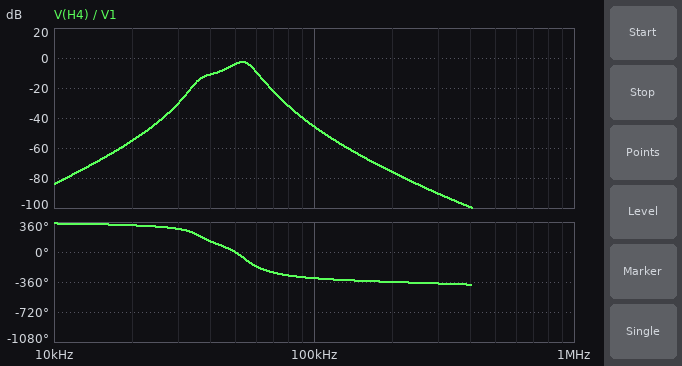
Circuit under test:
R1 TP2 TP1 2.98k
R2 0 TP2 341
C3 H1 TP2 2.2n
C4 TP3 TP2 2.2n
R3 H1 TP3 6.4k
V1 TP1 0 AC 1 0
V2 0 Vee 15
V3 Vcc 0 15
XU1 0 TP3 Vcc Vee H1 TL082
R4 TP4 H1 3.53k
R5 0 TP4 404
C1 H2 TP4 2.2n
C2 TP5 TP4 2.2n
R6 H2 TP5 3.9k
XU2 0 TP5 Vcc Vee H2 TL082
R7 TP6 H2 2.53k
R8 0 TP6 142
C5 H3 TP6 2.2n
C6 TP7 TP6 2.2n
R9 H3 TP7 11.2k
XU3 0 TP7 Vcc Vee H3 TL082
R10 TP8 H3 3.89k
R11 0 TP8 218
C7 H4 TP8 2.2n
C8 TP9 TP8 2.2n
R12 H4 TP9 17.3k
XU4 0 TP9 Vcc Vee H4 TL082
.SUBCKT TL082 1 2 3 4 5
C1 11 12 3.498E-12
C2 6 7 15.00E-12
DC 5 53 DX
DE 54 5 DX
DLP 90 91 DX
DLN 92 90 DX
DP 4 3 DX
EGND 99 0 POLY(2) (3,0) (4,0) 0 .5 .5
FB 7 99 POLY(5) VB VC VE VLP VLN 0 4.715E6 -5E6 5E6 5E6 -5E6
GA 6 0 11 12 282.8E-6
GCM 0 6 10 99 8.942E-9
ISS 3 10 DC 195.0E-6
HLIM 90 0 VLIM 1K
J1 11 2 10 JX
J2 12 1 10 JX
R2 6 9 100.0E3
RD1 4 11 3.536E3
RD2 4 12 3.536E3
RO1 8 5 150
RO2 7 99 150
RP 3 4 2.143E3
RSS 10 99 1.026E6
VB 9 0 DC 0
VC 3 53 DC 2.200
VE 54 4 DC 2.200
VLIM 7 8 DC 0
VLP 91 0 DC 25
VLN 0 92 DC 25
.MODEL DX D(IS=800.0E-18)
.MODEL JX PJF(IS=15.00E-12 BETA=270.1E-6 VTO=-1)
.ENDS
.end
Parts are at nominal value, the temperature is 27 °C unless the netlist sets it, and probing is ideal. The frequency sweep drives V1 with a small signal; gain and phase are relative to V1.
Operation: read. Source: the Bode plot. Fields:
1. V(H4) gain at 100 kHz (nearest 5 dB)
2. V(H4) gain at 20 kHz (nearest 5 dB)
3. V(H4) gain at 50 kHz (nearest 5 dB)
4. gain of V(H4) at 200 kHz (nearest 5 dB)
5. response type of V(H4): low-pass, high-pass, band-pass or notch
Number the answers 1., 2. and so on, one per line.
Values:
1. -45 dB
2. -55 dB
3. -5 dB
4. -75 dB
5. band-pass
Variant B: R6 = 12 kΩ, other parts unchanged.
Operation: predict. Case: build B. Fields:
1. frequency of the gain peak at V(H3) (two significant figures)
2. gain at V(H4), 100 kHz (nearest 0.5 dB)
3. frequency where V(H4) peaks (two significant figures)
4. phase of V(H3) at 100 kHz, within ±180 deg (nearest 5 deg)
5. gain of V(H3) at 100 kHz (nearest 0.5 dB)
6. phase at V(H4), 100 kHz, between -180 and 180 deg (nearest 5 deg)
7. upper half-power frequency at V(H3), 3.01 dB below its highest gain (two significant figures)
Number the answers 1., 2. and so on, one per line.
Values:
1. 53 kHz
2. -47.5 dB
3. 37 kHz
4. -65 deg
5. -33.0 dB
6. 25 deg
7. 57 kHz
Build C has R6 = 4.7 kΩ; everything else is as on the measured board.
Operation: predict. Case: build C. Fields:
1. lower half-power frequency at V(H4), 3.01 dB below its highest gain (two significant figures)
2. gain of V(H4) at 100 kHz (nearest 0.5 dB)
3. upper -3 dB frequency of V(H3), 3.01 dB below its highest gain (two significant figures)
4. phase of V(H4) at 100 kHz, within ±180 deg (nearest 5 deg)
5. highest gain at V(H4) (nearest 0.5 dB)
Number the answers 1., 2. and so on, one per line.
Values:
1. 47 kHz
2. -46.0 dB
3. 58 kHz
4. 40 deg
5. -0.5 dB
